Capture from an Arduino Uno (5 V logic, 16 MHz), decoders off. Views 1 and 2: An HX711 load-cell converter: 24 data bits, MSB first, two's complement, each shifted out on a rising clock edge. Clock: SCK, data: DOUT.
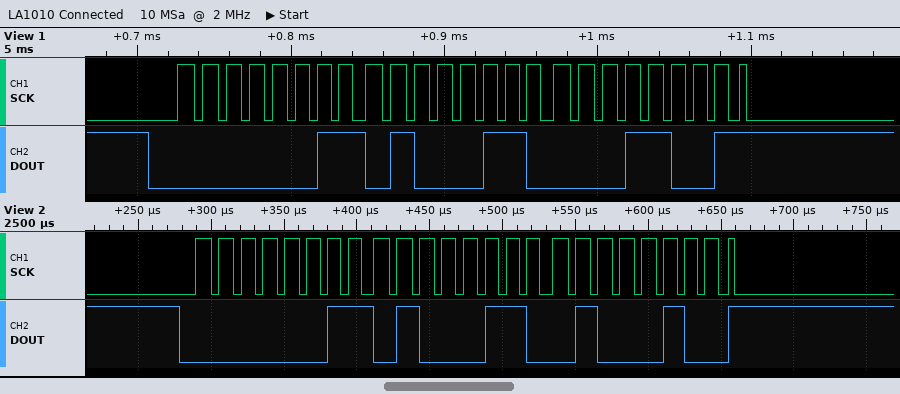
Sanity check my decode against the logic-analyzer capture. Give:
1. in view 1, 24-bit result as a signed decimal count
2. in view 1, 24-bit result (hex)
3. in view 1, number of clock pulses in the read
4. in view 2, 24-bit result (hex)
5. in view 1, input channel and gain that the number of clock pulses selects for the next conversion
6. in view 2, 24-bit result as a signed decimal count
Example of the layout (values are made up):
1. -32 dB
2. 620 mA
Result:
1. 214553
2. 0x034619
3. 25
4. 0x034644
5. channel A, gain 128
6. 214596
